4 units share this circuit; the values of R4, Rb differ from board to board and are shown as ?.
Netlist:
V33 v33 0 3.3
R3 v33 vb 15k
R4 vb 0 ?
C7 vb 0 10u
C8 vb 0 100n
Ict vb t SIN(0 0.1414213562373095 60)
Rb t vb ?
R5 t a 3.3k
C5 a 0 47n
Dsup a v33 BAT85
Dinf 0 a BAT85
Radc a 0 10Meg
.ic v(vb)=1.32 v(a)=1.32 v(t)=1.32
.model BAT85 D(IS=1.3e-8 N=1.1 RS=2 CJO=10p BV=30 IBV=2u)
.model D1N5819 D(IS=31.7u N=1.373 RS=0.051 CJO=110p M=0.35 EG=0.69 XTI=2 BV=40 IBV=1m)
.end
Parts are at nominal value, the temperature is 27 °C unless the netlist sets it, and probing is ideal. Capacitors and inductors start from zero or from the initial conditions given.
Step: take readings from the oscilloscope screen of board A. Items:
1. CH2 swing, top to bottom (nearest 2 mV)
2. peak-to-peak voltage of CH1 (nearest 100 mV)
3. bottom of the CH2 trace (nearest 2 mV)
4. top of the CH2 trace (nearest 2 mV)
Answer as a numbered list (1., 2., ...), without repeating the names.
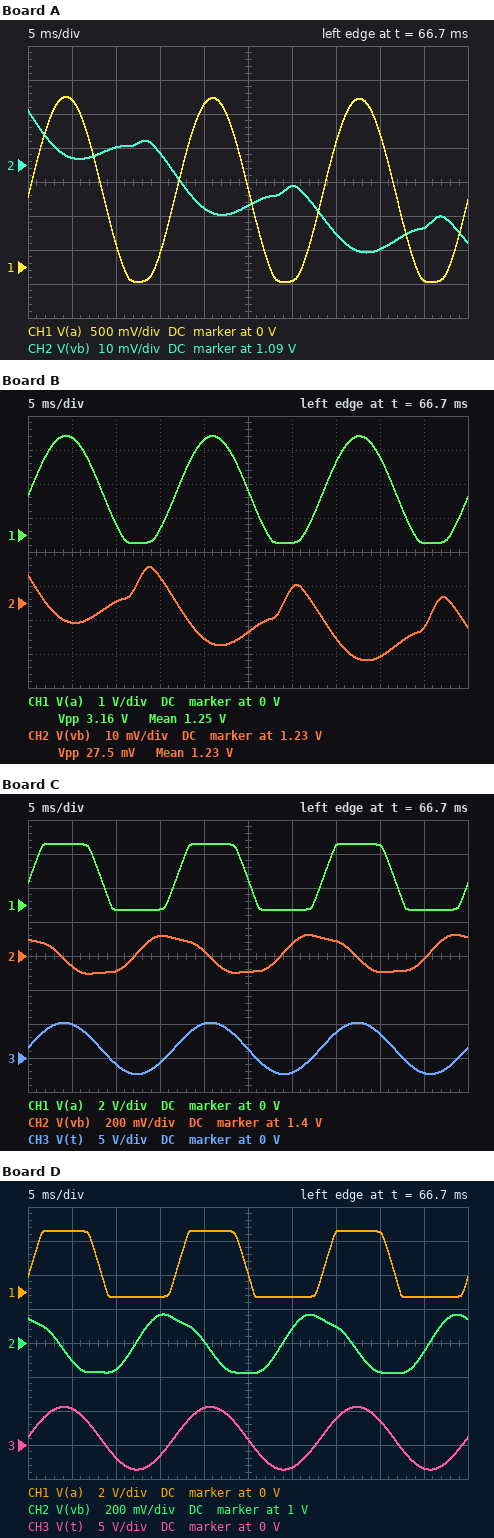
1. 42 mV
2. 2.7 V
3. 1.064 V
4. 1.106 V
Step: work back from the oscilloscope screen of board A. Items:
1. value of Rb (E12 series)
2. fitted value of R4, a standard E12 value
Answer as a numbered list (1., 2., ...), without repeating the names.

1. 10 Ω
2. 6.8 kΩ
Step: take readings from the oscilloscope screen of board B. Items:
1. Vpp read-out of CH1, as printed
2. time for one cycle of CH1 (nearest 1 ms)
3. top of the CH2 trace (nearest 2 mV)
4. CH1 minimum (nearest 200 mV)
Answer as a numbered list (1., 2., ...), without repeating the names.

1. 3.16 V
2. 17 ms
3. 1.240 V
4. -200 mV
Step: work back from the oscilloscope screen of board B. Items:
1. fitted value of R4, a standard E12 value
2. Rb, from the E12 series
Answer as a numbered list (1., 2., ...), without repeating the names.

1. 8.2 kΩ
2. 12 Ω
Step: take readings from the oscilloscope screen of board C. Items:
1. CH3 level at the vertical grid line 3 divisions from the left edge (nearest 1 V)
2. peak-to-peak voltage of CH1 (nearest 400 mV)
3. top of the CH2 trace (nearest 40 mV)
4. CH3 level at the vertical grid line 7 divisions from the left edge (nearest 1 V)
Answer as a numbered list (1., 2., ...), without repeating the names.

1. -1 V
2. 4.0 V
3. 1.52 V
4. 4 V
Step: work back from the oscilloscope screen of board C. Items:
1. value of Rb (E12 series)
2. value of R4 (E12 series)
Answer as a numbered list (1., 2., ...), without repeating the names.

1. 27 Ω
2. 8.2 kΩ
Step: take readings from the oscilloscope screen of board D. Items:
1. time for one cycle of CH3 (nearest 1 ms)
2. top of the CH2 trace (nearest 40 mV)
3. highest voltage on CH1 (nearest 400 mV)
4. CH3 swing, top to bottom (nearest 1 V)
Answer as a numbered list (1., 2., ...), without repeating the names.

1. 17 ms
2. 1.16 V
3. 3.6 V
4. 9 V
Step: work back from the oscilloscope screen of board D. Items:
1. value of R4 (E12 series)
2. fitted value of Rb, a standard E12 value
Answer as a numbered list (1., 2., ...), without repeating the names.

1. 3.3 kΩ
2. 33 Ω
